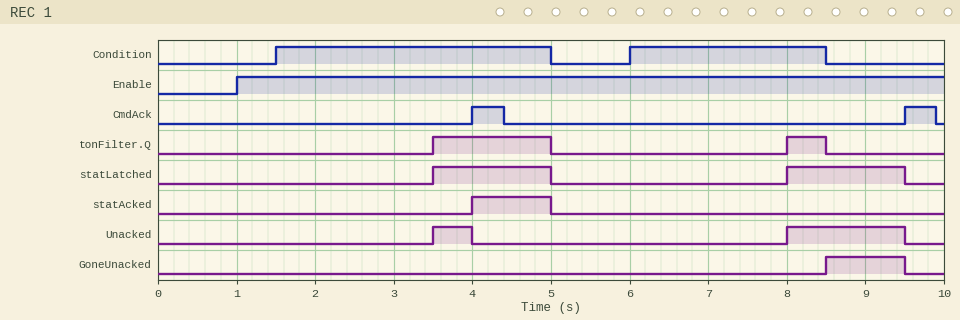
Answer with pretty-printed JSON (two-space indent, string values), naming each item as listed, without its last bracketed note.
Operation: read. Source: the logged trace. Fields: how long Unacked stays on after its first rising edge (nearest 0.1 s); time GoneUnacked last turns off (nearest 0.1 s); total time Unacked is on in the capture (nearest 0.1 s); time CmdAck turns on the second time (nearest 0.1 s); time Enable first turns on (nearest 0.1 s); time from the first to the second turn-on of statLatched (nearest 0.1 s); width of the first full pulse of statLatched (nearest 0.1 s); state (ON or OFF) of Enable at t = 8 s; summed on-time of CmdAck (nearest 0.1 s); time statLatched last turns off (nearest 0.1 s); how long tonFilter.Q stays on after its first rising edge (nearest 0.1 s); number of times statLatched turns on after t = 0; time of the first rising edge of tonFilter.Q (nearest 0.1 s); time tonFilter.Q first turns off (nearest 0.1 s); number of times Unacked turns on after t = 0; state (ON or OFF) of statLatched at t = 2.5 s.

{
  "how long Unacked stays on after its first rising edge": "0.5 s",
  "time GoneUnacked last turns off": "9.5 s",
  "total time Unacked is on in the capture": "2.0 s",
  "time CmdAck turns on the second time": "9.5 s",
  "time Enable first turns on": "1.0 s",
  "time from the first to the second turn-on of statLatched": "4.5 s",
  "width of the first full pulse of statLatched": "1.5 s",
  "state (ON or OFF) of Enable at t = 8 s": "ON",
  "summed on-time of CmdAck": "0.8 s",
  "time statLatched last turns off": "9.5 s",
  "how long tonFilter.Q stays on after its first rising edge": "1.5 s",
  "number of times statLatched turns on after t = 0": "2",
  "time of the first rising edge of tonFilter.Q": "3.5 s",
  "time tonFilter.Q first turns off": "5.0 s",
  "number of times Unacked turns on after t = 0": "2",
  "state (ON or OFF) of statLatched at t = 2.5 s": "OFF"
}
